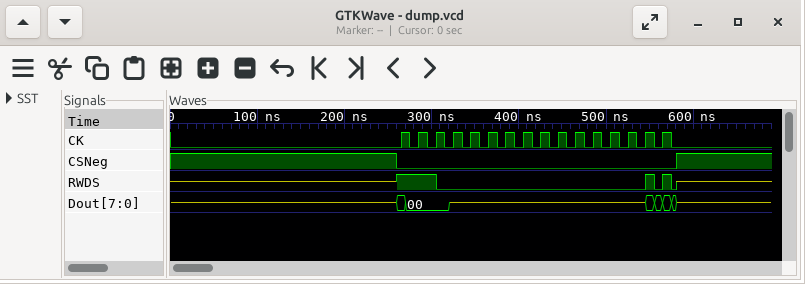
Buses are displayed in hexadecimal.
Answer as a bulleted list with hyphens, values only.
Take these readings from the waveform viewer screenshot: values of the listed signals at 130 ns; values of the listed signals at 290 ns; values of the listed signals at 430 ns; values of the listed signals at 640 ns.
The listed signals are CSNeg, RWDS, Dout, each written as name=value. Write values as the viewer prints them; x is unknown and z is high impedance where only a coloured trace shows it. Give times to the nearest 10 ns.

- CSNeg=1, RWDS=z, Dout=z
- CSNeg=0, RWDS=1, Dout=00
- CSNeg=0, RWDS=0, Dout=z
- CSNeg=1, RWDS=z, Dout=z
